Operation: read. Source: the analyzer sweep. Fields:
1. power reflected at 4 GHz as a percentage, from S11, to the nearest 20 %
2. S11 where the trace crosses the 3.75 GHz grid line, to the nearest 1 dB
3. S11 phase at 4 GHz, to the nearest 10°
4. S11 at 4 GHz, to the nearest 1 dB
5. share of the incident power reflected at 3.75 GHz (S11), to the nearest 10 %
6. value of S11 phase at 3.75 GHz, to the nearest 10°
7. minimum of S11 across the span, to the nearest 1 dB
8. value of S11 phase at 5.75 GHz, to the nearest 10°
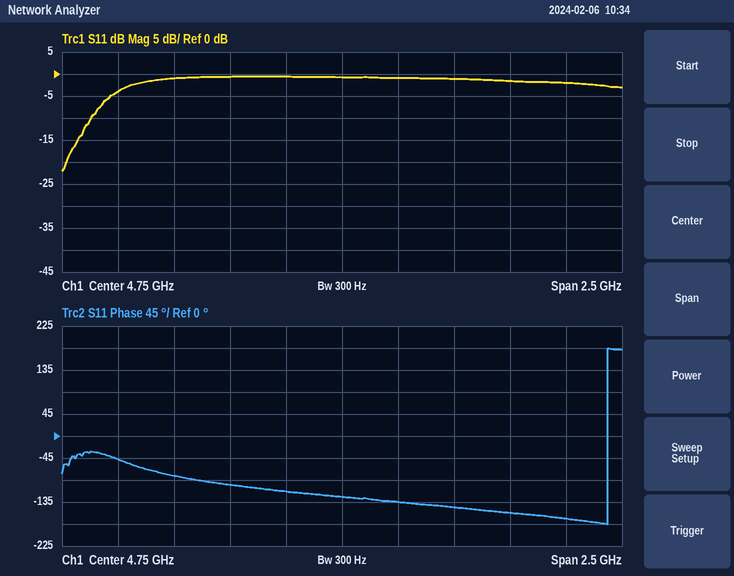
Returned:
80 %
-4 dB
-80°
-1 dB
40 %
-50°
-22 dB
-170°
